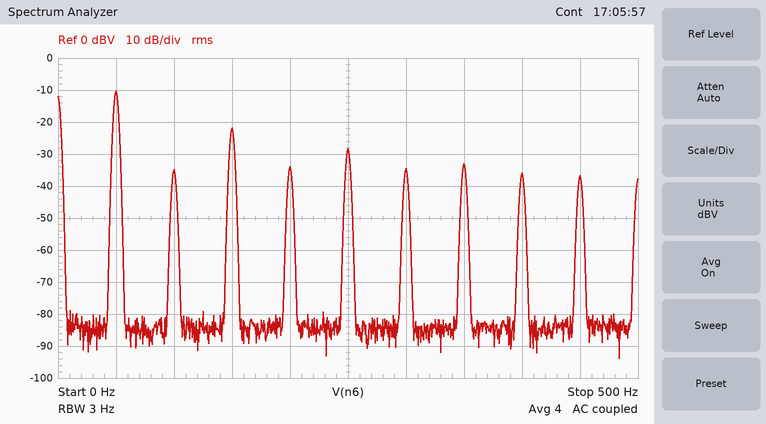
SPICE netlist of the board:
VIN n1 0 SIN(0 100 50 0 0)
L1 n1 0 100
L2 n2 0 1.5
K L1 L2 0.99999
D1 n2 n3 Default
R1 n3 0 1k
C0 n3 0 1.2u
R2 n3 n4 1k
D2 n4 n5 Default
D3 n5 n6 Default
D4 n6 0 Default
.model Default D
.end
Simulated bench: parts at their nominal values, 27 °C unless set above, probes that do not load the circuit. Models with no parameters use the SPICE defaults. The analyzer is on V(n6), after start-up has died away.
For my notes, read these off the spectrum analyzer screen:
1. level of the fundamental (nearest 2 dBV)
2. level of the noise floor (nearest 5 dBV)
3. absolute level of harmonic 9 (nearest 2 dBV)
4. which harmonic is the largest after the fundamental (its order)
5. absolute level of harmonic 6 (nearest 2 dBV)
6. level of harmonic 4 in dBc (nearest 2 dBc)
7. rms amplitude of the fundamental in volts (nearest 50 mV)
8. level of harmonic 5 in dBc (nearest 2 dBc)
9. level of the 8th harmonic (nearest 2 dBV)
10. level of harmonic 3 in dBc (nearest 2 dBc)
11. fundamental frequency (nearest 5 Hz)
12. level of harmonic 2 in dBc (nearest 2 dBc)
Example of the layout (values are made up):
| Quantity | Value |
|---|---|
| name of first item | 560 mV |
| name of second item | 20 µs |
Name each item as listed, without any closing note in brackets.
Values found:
| Quantity | Value |
|---|---|
| level of the fundamental | -10 dBV |
| level of the noise floor | -85 dBV |
| absolute level of harmonic 9 | -36 dBV |
| which harmonic is the largest after the fundamental | 3 |
| absolute level of harmonic 6 | -34 dBV |
| level of harmonic 4 in dBc | -24 dBc |
| rms amplitude of the fundamental in volts | 300 mV |
| level of harmonic 5 in dBc | -18 dBc |
| level of the 8th harmonic | -36 dBV |
| level of harmonic 3 in dBc | -12 dBc |
| fundamental frequency | 50 Hz |
| level of harmonic 2 in dBc | -24 dBc |
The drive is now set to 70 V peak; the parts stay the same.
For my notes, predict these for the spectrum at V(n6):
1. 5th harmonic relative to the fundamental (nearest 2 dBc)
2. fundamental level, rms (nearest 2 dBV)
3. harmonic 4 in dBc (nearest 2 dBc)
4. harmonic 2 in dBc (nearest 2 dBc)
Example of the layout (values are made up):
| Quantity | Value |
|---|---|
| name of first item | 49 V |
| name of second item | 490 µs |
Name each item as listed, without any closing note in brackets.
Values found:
| Quantity | Value |
|---|---|
| 5th harmonic relative to the fundamental | -20 dBc |
| fundamental level, rms | -10 dBV |
| harmonic 4 in dBc | -20 dBc |
| harmonic 2 in dBc | -18 dBc |
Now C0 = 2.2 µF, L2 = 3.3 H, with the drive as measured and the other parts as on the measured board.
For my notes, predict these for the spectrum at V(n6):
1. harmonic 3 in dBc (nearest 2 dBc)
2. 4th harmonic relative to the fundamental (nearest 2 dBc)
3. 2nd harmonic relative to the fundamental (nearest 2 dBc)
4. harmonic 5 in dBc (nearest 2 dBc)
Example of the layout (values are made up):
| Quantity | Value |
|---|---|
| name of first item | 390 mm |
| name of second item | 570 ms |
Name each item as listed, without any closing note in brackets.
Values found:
| Quantity | Value |
|---|---|
| harmonic 3 in dBc | -14 dBc |
| 4th harmonic relative to the fundamental | -18 dBc |
| 2nd harmonic relative to the fundamental | -12 dBc |
| harmonic 5 in dBc | -20 dBc |
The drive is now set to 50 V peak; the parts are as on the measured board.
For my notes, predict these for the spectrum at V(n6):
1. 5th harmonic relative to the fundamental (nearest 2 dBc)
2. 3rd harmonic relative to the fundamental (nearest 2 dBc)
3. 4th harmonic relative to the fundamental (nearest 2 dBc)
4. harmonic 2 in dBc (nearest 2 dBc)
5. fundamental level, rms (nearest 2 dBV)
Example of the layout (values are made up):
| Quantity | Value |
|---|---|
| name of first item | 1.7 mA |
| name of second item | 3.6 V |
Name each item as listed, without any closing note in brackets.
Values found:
| Quantity | Value |
|---|---|
| 5th harmonic relative to the fundamental | -24 dBc |
| 3rd harmonic relative to the fundamental | -14 dBc |
| 4th harmonic relative to the fundamental | -16 dBc |
| harmonic 2 in dBc | -14 dBc |
| fundamental level, rms | -10 dBV |
